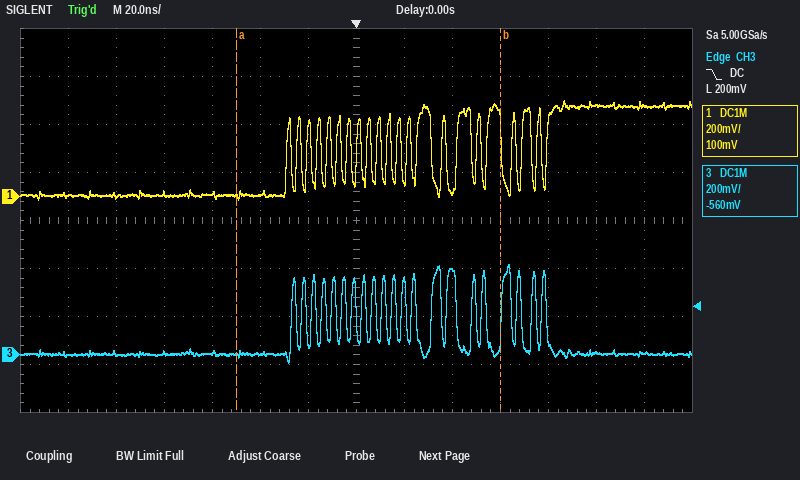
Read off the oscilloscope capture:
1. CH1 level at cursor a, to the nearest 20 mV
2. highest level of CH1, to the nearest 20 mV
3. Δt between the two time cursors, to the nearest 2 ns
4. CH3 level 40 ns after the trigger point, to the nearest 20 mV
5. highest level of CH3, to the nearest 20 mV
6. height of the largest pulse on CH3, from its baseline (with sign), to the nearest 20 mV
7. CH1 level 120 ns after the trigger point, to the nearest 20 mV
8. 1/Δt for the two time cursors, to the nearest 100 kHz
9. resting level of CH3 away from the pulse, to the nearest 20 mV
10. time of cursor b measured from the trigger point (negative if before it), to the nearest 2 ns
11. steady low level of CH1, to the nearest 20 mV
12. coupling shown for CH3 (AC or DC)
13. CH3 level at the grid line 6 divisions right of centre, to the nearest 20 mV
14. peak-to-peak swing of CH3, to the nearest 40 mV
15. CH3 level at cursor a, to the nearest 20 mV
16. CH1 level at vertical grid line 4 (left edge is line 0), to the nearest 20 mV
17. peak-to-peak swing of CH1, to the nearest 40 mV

0 mV
400 mV
110 ns
360 mV
380 mV
+380 mV
380 mV
9.1 MHz
0 mV
+60 ns
0 mV
DC
0 mV
400 mV
0 mV
20 mV
400 mV
